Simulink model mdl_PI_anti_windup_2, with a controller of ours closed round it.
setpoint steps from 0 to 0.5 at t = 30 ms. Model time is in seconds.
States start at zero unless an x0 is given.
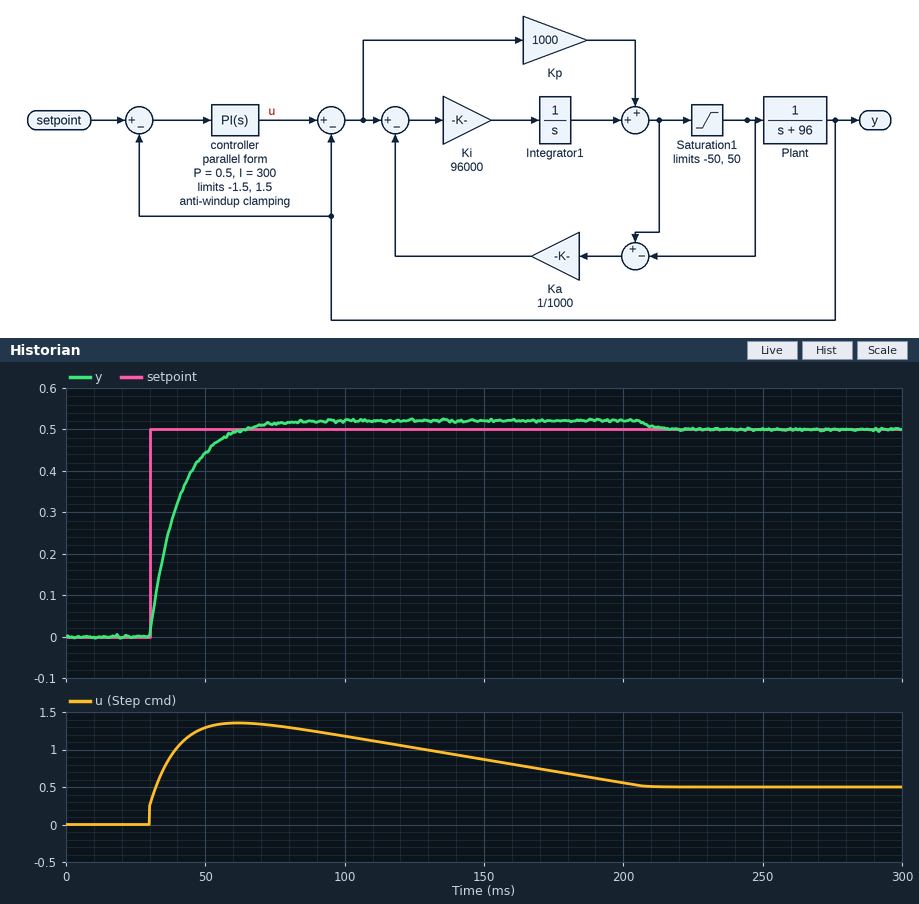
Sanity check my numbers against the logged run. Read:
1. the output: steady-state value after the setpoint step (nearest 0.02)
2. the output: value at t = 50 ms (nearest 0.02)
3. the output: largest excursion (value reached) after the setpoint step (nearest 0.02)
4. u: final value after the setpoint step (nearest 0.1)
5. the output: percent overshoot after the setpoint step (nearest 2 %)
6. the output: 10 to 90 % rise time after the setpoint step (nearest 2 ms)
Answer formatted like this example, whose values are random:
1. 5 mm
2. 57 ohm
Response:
1. 0.50
2. 0.44
3. 0.52
4. 0.5
5. 4 %
6. 20 ms
